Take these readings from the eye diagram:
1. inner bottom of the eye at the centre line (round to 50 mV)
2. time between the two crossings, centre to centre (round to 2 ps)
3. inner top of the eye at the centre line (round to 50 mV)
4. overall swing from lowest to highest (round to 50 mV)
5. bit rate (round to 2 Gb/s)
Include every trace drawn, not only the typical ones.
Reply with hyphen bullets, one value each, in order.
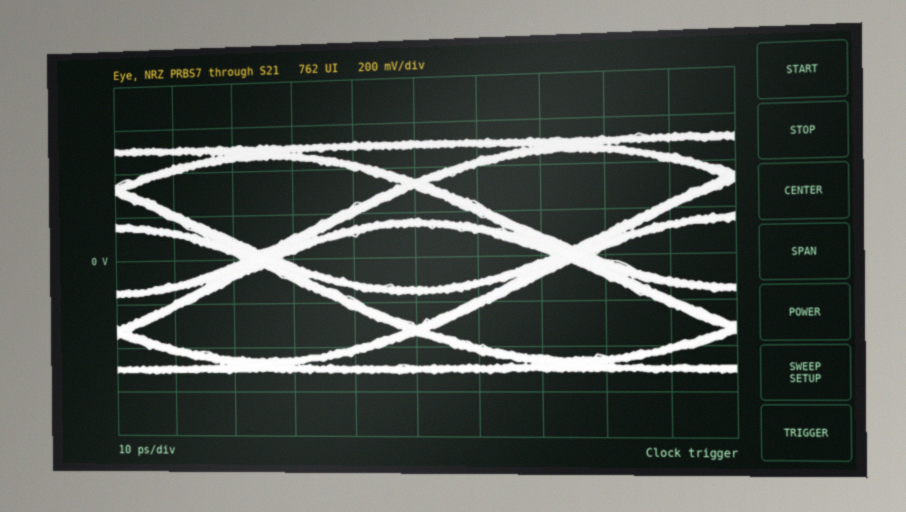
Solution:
- -150 mV
- 50 ps
- 150 mV
- 1.05 V
- 20 Gb/s
